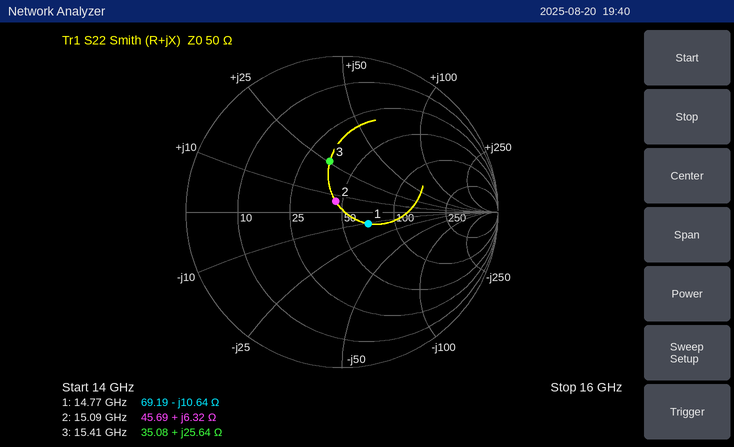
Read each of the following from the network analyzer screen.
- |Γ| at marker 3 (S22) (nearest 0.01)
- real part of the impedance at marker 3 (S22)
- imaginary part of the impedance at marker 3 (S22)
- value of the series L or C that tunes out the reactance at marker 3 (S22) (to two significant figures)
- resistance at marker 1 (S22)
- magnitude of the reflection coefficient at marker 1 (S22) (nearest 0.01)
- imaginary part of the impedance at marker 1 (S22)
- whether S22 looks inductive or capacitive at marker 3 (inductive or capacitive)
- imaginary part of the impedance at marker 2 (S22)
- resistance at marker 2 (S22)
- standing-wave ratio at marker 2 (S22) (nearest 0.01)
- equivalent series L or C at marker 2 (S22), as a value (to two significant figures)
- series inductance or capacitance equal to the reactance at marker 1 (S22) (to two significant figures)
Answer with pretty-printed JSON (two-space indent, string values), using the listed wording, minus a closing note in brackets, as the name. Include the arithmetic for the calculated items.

{
  "|Γ| at marker 3 (S22)": "0.33",
  "real part of the impedance at marker 3": "35.08 Ω",
  "imaginary part of the impedance at marker 3": "+25.64 Ω",
  "value of the series L or C that tunes out the reactance at marker 3 (S22)": "C = 1/(2π × 15.41 GHz × 25.64 Ω) ≈ 403 fF, so 400 fF to two significant figures",
  "resistance at marker 1": "69.19 Ω",
  "magnitude of the reflection coefficient at marker 1 (S22)": "0.18",
  "imaginary part of the impedance at marker 1": "-10.64 Ω",
  "whether S22 looks inductive or capacitive at marker 3": "inductive",
  "imaginary part of the impedance at marker 2": "+6.32 Ω",
  "resistance at marker 2": "45.69 Ω",
  "standing-wave ratio at marker 2 (S22)": "1.17",
  "equivalent series L or C at marker 2 (S22), as a value": "L = 6.32 Ω/(2π × 15.09 GHz) ≈ 67 pH",
  "series inductance or capacitance equal to the reactance at marker 1 (S22)": "C = 1/(2π × 14.77 GHz × 10.64 Ω) ≈ 1.0 pF"
}
